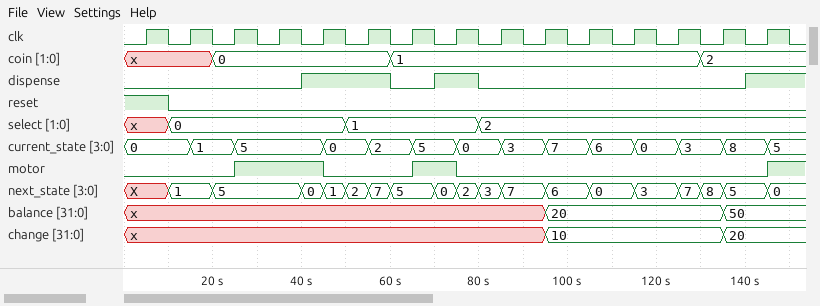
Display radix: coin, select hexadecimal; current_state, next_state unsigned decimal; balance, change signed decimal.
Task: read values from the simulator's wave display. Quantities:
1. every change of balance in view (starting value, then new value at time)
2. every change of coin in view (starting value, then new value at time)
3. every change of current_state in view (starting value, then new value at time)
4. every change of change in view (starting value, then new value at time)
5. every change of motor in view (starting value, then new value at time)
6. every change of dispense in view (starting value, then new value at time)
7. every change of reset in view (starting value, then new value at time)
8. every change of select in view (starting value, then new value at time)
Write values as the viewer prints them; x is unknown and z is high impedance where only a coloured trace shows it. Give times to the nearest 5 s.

x, 20 at 95 s, 50 at 135 s
x, 0 at 20 s, 1 at 60 s, 2 at 130 s
0, 1 at 15 s, 5 at 25 s, 0 at 45 s, 2 at 55 s, 5 at 65 s, 0 at 75 s, 3 at 85 s, 7 at 95 s, 6 at 105 s, 0 at 115 s, 3 at 125 s, 8 at 135 s, 5 at 145 s
x, 10 at 95 s, 20 at 135 s
0, 1 at 25 s, 0 at 45 s, 1 at 65 s, 0 at 75 s, 1 at 145 s
0, 1 at 40 s, 0 at 60 s, 1 at 70 s, 0 at 80 s, 1 at 140 s
1, 0 at 10 s
x, 0 at 10 s, 1 at 50 s, 2 at 80 s
